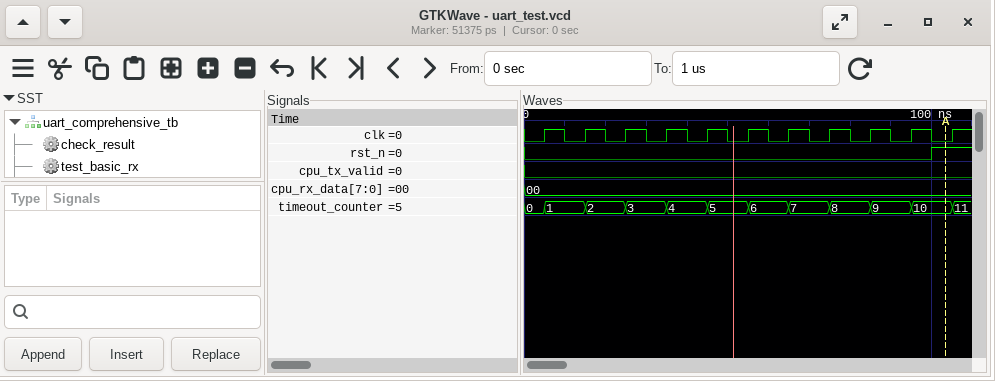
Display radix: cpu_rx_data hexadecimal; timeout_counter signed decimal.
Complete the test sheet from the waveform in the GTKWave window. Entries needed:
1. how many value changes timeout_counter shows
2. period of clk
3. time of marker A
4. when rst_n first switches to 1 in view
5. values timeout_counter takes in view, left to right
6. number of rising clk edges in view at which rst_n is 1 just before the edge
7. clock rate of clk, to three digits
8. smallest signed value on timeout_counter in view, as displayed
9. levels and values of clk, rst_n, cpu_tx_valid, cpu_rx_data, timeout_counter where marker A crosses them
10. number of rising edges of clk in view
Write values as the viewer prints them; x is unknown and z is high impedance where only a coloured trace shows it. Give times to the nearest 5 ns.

11
10 ns
105 ns
100 ns
0, 1, 2, 3, 4, 5, 6, 7, 8, 9, 10, 11
1
100 MHz
0
clk=0, rst_n=1, cpu_tx_valid=0, cpu_rx_data=00, timeout_counter=10
11
